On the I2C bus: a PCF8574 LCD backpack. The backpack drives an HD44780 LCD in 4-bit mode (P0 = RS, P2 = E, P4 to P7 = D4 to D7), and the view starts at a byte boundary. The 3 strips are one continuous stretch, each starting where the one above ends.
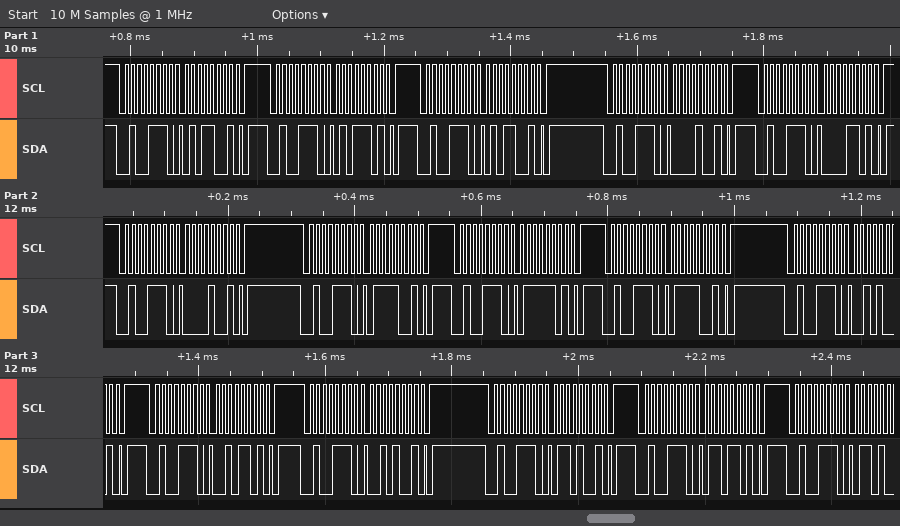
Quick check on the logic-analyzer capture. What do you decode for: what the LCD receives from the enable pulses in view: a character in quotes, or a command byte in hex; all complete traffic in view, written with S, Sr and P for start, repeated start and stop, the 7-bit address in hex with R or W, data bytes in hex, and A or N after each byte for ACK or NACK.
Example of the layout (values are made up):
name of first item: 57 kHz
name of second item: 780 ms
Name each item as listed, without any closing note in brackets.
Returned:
what the LCD receives from the enable pulses in view: a character in quotes, or a command byte in hex: 'P' 'r'
all complete traffic in view, written with S, Sr and P for start, repeated start and stop, the 7-bit address in hex with R or W, data bytes in hex, and A or N after each byte for ACK or NACK: S 27W A 59 A P S 27W A 5D A P S 27W A 59 A P S 27W A 09 A P S 27W A 0D A P S 27W A 09 A P S 27W A 79 A P S 27W A 7D A P S 27W A 79 A P S 27W A 29 A P S 27W A 2D A P S 27W A 29 A P S 27W A 69 A P S 27W A 6D A P S 27W A
